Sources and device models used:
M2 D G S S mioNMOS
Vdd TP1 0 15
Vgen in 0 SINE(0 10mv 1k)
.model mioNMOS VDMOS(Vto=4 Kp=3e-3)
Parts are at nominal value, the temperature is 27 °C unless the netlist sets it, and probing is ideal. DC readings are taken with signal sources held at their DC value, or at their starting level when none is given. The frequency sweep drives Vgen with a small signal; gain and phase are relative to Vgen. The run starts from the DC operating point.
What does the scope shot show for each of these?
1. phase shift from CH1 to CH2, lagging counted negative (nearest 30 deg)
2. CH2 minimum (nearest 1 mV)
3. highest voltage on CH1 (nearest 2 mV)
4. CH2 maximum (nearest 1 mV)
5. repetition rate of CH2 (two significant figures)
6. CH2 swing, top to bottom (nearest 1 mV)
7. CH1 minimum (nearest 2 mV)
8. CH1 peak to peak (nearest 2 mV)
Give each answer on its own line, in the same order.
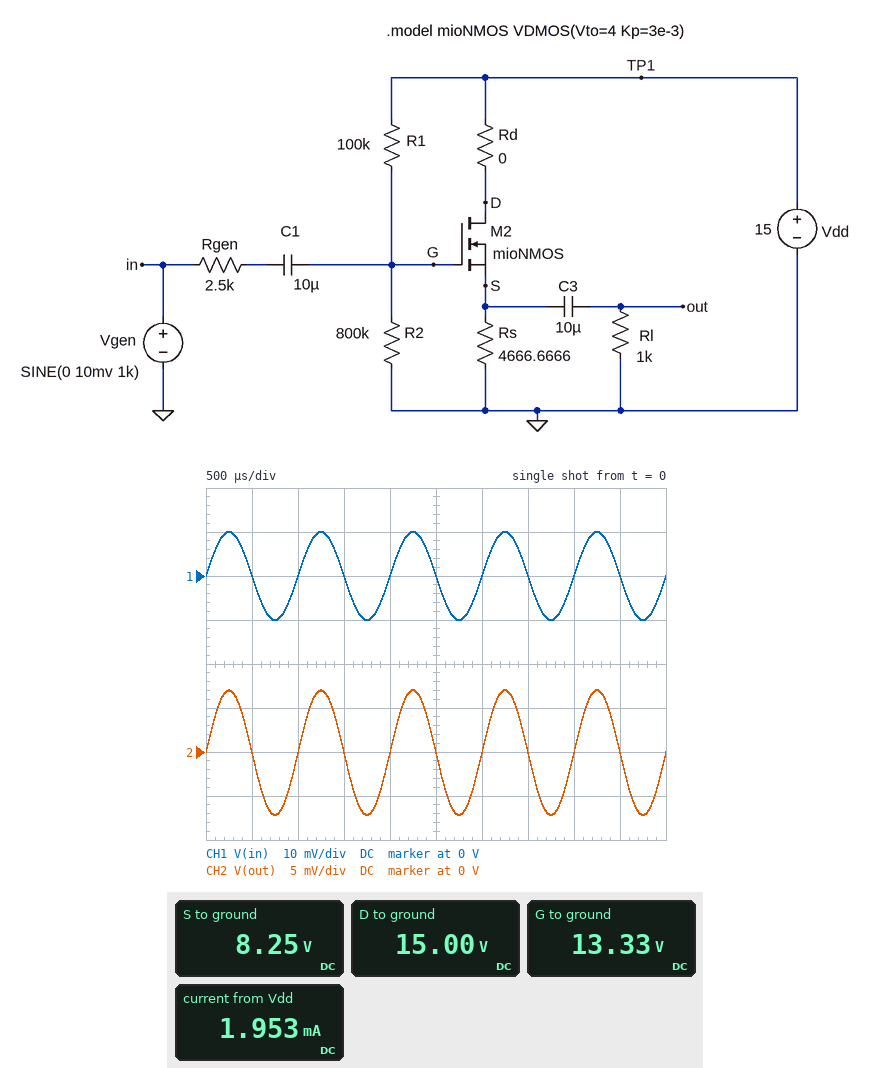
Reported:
0 deg
-7 mV
10 mV
7 mV
1.0 kHz
14 mV
-10 mV
20 mV
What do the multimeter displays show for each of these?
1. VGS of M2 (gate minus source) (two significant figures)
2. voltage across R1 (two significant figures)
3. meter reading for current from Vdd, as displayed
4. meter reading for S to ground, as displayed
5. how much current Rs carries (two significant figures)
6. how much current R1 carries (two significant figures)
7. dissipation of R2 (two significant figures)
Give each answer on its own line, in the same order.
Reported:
5.1 V
1.7 V
1.953 mA
8.25 V
1.8 mA
17 µA
220 µW
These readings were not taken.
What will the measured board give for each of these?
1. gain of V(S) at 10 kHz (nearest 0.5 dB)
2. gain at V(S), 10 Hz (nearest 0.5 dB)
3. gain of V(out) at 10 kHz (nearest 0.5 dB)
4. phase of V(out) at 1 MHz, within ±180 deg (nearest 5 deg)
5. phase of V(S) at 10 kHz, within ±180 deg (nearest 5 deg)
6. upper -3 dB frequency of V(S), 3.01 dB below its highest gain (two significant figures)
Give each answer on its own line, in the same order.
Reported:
-3.0 dB
-1.5 dB
-3.0 dB
-70 deg
-5 deg
37 kHz
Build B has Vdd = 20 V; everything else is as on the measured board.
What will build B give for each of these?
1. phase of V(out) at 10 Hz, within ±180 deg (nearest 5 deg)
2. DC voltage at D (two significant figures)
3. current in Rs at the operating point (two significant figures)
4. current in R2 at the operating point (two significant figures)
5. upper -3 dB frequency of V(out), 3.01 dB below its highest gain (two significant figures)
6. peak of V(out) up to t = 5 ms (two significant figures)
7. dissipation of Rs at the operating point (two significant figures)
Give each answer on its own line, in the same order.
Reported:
55 deg
20 V
2.7 mA
22 µA
95 kHz
7.4 mV
33 mW
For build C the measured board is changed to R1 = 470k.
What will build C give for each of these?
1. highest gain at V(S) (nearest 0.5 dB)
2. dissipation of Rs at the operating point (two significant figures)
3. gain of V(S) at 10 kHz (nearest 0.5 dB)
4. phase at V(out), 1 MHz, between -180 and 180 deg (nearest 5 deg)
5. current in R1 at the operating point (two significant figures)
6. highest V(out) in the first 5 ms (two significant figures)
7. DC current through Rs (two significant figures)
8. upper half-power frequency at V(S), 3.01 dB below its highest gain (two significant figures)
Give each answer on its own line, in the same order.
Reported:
-1.0 dB
4.6 mW
-3.5 dB
-55 deg
12 µA
6.6 mV
990 µA
23 kHz
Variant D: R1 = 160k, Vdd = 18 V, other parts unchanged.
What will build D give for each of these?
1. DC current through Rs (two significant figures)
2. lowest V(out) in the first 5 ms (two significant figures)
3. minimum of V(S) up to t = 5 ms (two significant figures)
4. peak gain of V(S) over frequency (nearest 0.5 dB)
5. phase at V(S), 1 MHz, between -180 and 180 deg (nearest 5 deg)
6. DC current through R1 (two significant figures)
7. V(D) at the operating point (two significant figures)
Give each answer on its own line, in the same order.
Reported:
2.1 mA
-7.4 mV
9.8 V
-0.5 dB
-65 deg
19 µA
18 V
